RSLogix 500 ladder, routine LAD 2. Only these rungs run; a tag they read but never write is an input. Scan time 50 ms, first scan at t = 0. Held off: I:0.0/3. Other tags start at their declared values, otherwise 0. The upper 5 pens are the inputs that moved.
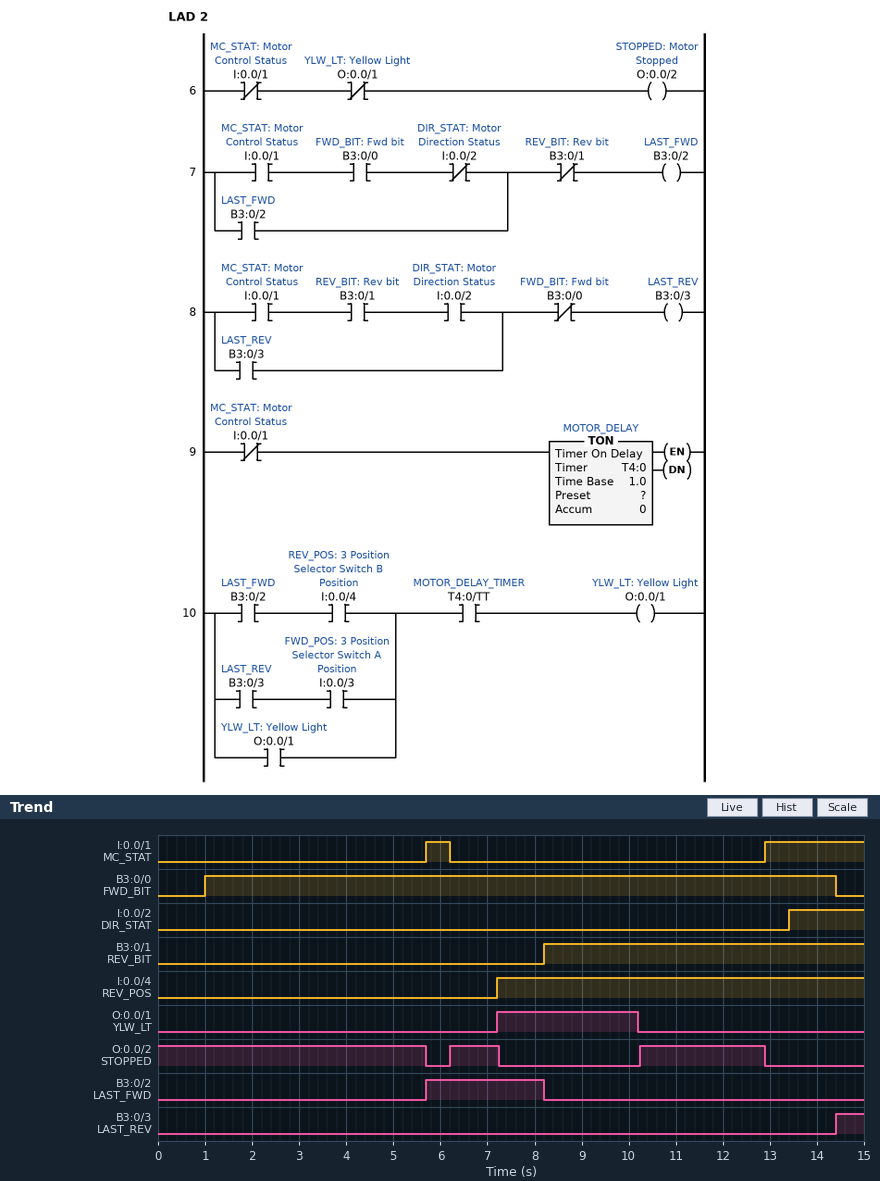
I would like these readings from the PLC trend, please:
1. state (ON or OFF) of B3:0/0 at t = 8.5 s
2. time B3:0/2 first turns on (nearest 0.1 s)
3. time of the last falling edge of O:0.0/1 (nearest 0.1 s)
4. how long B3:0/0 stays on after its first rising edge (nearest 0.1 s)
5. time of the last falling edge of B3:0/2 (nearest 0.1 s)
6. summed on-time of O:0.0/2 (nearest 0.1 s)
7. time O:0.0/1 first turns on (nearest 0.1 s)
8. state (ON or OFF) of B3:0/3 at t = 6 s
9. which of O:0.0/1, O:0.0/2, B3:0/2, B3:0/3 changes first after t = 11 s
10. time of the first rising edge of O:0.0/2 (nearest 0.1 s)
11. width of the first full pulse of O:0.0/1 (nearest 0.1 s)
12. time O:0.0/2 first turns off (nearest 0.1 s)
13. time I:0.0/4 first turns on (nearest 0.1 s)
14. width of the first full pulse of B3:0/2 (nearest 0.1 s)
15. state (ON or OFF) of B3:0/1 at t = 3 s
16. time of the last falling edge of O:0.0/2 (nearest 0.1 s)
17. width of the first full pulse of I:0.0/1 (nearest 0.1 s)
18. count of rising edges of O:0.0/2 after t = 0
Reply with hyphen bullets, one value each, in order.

- ON
- 5.7 s
- 10.2 s
- 13.4 s
- 8.2 s
- 9.4 s
- 7.2 s
- OFF
- O:0.0/2
- 6.2 s
- 3.0 s
- 5.7 s
- 7.2 s
- 2.5 s
- OFF
- 12.9 s
- 0.5 s
- 2
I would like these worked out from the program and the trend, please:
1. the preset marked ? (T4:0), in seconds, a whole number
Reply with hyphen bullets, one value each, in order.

- 4 s
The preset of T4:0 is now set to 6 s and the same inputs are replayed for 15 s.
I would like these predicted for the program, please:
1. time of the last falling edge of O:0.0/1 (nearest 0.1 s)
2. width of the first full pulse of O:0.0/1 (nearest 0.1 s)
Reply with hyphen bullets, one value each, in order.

- 12.2 s
- 5.0 s
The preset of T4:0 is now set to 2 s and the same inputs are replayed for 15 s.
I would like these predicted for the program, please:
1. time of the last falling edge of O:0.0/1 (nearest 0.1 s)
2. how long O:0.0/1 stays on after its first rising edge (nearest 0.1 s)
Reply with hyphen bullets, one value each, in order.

- 8.2 s
- 1.0 s
